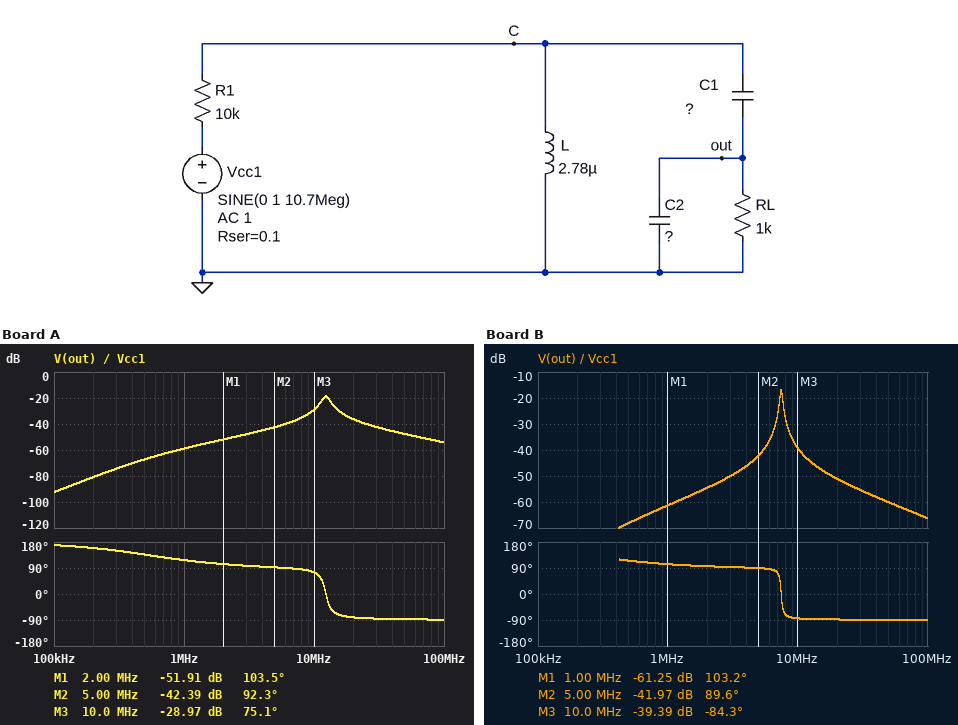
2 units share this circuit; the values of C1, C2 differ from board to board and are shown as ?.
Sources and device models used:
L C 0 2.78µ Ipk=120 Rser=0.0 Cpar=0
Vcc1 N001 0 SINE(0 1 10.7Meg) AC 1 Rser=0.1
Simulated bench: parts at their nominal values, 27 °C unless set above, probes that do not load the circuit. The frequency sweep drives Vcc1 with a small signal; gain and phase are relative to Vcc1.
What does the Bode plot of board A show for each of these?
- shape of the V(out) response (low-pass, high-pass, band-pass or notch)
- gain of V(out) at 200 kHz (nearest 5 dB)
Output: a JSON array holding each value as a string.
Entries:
["band-pass", "-80 dB"]
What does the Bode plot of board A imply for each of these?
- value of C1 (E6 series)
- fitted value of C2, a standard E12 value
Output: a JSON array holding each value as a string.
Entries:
["220 pF", "82 pF"]
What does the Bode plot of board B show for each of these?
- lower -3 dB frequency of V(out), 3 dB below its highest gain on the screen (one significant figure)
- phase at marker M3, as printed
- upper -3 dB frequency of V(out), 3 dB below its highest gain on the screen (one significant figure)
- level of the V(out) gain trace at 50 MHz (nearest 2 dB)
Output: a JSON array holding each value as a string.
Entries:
["7 MHz", "-84.3 deg", "8 MHz", "-60 dB"]
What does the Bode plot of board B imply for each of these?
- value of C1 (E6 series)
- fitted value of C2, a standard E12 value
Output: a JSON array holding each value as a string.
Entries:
["330 pF", "330 pF"]
